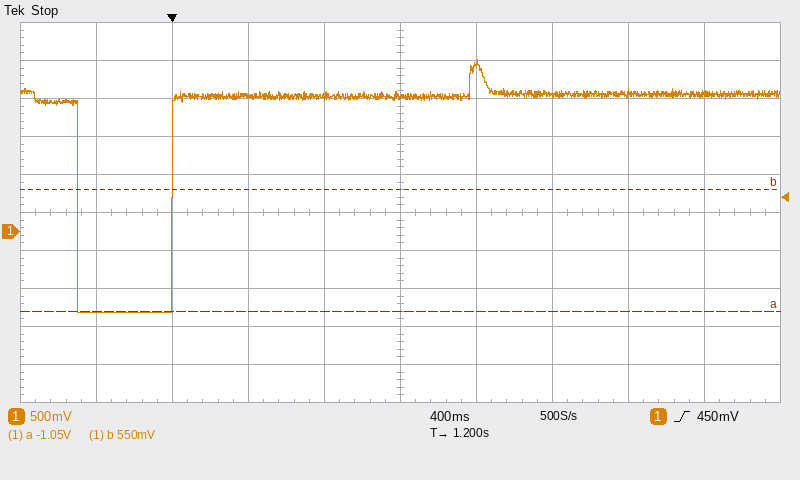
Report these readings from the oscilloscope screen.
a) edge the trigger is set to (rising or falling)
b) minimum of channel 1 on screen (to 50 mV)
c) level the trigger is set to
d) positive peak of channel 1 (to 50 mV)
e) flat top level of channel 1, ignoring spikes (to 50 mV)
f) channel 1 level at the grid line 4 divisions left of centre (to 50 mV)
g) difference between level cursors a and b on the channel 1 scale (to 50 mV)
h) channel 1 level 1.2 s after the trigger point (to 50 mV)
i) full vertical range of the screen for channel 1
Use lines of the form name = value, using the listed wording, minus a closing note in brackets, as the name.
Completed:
edge the trigger is set to = rising
minimum of channel 1 on screen = -1.05 V
level the trigger is set to = 450 mV
positive peak of channel 1 = 2.25 V
flat top level of channel 1, ignoring spikes = 1.80 V
channel 1 level at the grid line 4 divisions left of centre = -1.05 V
difference between level cursors a and b on the channel 1 scale = 1.60 V
channel 1 level 1.2 s after the trigger point = 1.80 V
full vertical range of the screen for channel 1 = 5 V
